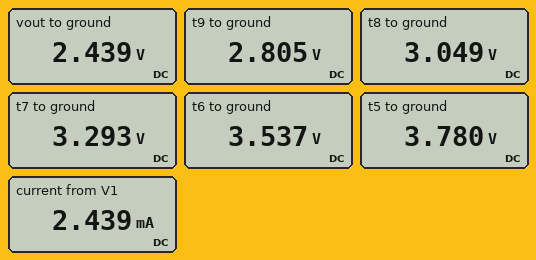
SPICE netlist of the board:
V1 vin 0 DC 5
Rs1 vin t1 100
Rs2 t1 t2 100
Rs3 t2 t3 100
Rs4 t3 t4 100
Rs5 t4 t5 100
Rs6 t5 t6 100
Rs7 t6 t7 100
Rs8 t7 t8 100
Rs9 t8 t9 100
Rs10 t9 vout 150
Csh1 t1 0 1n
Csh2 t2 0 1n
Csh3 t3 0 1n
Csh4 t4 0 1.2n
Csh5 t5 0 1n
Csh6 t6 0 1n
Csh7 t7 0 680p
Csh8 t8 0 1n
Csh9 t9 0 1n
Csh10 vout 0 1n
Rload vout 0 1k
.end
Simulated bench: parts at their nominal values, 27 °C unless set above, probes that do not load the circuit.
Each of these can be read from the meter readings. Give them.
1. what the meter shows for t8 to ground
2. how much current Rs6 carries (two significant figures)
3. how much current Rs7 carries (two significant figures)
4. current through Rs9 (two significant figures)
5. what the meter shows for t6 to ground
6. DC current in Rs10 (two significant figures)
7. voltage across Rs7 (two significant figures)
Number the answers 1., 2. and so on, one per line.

1. 3.049 V
2. 2.4 mA
3. 2.4 mA
4. 2.4 mA
5. 3.537 V
6. 2.4 mA
7. 240 mV
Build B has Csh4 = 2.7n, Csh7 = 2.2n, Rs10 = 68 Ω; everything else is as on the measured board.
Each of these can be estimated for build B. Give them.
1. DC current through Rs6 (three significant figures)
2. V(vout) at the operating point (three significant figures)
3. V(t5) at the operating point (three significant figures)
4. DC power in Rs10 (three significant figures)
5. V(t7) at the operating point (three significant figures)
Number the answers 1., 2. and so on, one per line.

1. 2.54 mA
2. 2.54 V
3. 3.73 V
4. 439 µW
5. 3.22 V
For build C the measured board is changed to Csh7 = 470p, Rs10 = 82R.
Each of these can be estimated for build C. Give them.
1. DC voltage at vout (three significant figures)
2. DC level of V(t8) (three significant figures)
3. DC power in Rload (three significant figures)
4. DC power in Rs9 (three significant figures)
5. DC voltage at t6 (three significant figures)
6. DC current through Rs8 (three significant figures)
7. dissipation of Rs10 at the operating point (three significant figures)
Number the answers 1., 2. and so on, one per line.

1. 2.52 V
2. 2.98 V
3. 6.36 mW
4. 636 µW
5. 3.49 V
6. 2.52 mA
7. 522 µW
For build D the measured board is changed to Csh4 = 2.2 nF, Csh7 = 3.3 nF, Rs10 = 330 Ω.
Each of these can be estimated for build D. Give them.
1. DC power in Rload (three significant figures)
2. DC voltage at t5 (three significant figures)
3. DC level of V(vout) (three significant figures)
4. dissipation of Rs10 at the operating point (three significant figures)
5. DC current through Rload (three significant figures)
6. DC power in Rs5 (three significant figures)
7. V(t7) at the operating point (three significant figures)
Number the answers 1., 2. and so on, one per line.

1. 5.03 mW
2. 3.88 V
3. 2.24 V
4. 1.66 mW
5. 2.24 mA
6. 503 µW
7. 3.43 V
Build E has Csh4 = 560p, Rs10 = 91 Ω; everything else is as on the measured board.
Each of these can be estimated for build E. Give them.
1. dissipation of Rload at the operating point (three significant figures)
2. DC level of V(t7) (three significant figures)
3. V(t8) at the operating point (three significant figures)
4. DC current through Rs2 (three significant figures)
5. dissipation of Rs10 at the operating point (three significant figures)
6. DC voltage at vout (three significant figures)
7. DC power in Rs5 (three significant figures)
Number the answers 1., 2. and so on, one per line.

1. 6.31 mW
2. 3.24 V
3. 2.99 V
4. 2.51 mA
5. 574 µW
6. 2.51 V
7. 631 µW
